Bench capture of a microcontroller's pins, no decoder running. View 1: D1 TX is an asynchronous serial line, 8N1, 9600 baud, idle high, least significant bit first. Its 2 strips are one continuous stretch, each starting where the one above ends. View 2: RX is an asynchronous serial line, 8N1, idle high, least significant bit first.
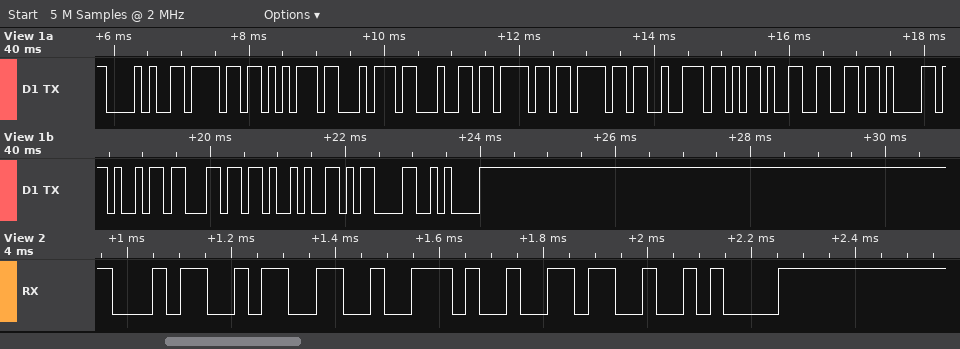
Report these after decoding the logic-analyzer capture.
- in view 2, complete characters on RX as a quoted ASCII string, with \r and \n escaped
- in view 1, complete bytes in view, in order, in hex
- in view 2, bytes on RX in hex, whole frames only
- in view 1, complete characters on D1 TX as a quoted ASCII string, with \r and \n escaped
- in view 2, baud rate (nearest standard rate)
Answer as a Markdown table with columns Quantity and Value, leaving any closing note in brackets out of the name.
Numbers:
| Quantity | Value |
|---|---|
| in view 2, complete characters on RX as a quoted ASCII string, with \r and \n escaped | "43.6\n" |
| in view 1, complete bytes in view, in order, in hex | 28 6F 75 74 64 6F 6F 72 2D 66 61 69 6C 29 0D 0A |
| in view 2, bytes on RX in hex, whole frames only | 34 33 2E 36 0A |
| in view 1, complete characters on D1 TX as a quoted ASCII string, with \r and \n escaped | "(outdoor-fail)\r\n" |
| in view 2, baud rate | 38400 baud |
